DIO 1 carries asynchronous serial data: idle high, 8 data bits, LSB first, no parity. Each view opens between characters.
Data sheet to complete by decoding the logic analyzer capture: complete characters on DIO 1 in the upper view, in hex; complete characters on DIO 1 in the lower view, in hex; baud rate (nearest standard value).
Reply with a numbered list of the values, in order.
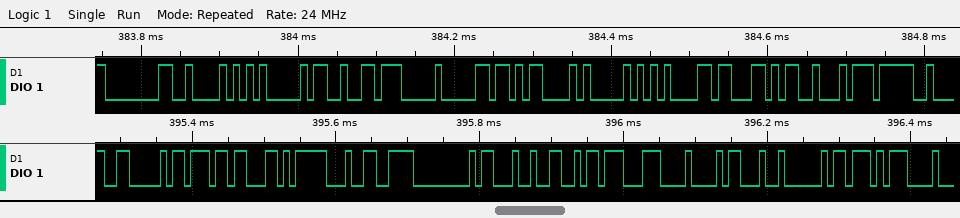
1. 80, 42, 05, 93, 07, B0, 0D, 41, 85, 63, 13, F7
2. 06, BB, 63, 1F, E6, 00, 23, A6, C7, 08, 23, A0, D7
3. 115200 baud
